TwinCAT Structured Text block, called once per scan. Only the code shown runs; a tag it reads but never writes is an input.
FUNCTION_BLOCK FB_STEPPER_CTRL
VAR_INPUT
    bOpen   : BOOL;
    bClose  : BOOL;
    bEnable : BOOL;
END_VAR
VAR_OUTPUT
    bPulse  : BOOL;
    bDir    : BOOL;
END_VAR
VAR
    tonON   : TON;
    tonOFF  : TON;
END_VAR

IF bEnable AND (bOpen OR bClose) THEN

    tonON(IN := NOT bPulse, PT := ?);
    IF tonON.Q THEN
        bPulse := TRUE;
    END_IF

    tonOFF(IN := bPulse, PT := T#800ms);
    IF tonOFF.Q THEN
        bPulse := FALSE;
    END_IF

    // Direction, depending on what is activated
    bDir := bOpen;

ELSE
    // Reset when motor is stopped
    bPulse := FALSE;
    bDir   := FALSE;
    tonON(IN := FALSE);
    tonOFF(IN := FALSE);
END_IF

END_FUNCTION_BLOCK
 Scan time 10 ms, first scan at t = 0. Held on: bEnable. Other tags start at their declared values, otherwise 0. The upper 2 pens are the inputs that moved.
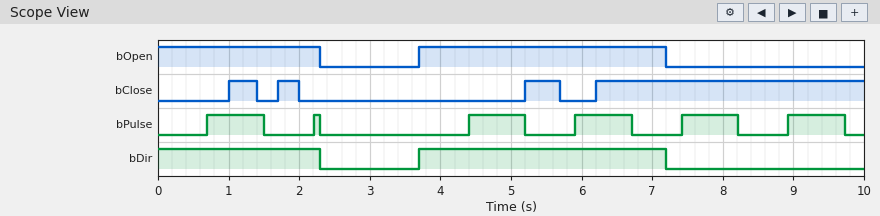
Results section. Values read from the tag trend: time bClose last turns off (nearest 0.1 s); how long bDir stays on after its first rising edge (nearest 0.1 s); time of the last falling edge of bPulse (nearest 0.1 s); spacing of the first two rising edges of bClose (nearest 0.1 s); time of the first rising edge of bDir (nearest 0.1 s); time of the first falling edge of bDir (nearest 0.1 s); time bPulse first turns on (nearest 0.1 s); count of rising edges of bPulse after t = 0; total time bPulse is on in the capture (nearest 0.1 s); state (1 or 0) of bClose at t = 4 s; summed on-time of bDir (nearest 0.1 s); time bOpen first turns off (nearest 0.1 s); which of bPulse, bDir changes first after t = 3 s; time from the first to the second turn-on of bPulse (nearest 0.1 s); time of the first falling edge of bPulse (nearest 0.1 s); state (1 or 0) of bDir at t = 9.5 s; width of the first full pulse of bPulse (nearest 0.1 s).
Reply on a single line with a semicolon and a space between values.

5.7 s; 3.5 s; 9.7 s; 0.7 s; 3.7 s; 2.3 s; 0.7 s; 6; 4.1 s; 0; 5.8 s; 2.3 s; bDir; 1.5 s; 1.5 s; 0; 0.8 s
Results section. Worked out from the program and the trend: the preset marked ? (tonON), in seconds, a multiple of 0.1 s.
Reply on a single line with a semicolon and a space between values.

0.7 s
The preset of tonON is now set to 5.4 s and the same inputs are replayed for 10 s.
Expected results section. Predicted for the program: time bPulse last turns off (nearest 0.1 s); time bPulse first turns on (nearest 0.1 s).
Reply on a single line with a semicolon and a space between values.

9.9 s; 9.1 s
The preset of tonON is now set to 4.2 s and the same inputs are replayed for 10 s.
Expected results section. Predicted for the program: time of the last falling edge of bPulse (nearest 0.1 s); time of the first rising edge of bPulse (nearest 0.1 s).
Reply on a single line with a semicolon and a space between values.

8.7 s; 7.9 s
